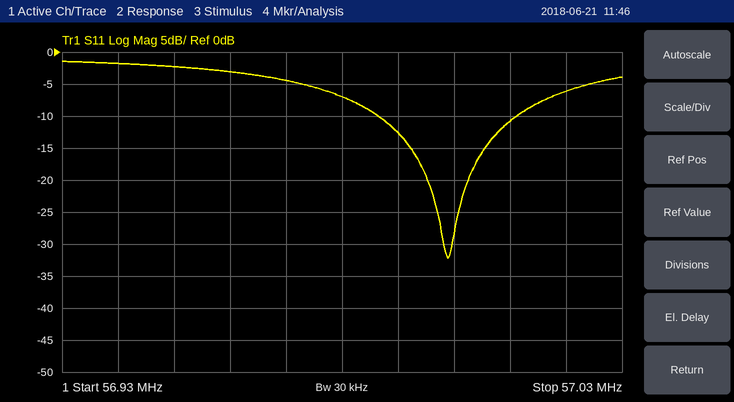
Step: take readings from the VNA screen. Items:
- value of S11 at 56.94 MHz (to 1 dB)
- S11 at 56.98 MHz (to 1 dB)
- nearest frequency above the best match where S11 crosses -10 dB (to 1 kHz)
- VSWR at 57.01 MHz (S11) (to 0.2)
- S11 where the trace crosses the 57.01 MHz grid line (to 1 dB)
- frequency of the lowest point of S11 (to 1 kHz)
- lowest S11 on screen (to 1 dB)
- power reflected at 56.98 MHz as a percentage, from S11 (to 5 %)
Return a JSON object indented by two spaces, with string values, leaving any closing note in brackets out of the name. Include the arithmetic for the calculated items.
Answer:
{
  "value of S11 at 56.94 MHz": "-2 dB",
  "S11 at 56.98 MHz": "-7 dB",
  "nearest frequency above the best match where S11 crosses -10 dB": "57.011 MHz",
  "VSWR at 57.01 MHz (S11)": "|Γ| = 10^(-11/20) = 0.2818; VSWR = (1 + 0.2818)/(1 − 0.2818) ≈ 1.8",
  "S11 where the trace crosses the 57.01 MHz grid line": "-11 dB",
  "frequency of the lowest point of S11": "56.999 MHz",
  "lowest S11 on screen": "-32 dB",
  "power reflected at 56.98 MHz as a percentage, from S11": "10^(-7/10) ≈ 20 %"
}
